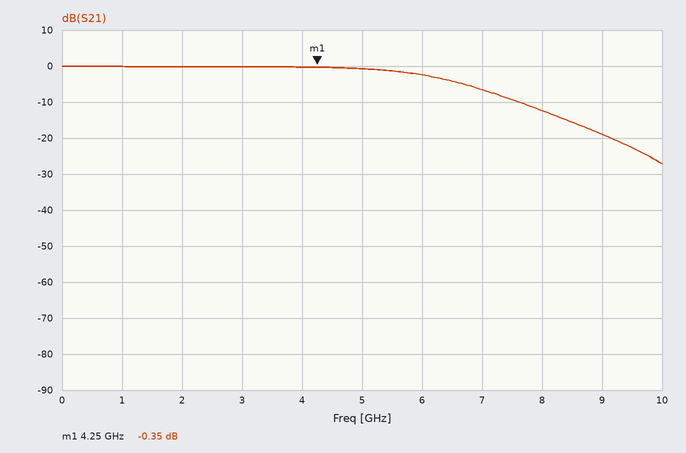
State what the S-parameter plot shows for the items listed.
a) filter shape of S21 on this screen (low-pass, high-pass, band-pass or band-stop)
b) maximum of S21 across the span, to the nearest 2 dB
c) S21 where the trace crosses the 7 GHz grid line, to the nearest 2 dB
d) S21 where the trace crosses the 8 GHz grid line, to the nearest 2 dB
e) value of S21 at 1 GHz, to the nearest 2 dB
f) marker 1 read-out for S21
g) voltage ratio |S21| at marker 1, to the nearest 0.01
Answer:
low-pass
0 dB
-6 dB
-12 dB
0 dB
-0.35 dB
0.96
